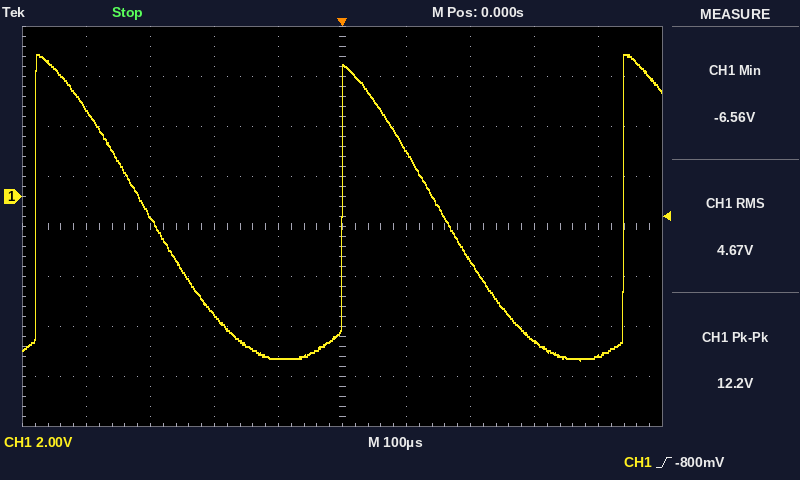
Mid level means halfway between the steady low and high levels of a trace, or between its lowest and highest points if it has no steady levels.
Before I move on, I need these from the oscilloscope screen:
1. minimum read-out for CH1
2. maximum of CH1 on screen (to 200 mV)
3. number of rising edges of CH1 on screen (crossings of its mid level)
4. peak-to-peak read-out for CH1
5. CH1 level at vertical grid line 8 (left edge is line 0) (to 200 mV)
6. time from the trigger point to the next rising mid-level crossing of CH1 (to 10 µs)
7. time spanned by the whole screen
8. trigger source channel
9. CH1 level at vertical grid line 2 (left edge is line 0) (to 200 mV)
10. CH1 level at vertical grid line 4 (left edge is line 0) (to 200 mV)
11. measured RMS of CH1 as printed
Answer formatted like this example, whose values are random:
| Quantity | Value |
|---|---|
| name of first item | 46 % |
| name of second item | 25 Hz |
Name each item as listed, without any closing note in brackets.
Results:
| Quantity | Value |
|---|---|
| minimum read-out for CH1 | -6.56 V |
| maximum of CH1 on screen | 5.6 V |
| number of rising edges of CH1 on screen | 3 |
| peak-to-peak read-out for CH1 | 12.2 V |
| CH1 level at vertical grid line 8 (left edge is line 0) | -5.8 V |
| time from the trigger point to the next rising mid-level crossing of CH1 | 440 µs |
| time spanned by the whole screen | 1 ms |
| trigger source channel | CH1 |
| CH1 level at vertical grid line 2 (left edge is line 0) | -800 mV |
| CH1 level at vertical grid line 4 (left edge is line 0) | -6.4 V |
| measured RMS of CH1 as printed | 4.67 V |
